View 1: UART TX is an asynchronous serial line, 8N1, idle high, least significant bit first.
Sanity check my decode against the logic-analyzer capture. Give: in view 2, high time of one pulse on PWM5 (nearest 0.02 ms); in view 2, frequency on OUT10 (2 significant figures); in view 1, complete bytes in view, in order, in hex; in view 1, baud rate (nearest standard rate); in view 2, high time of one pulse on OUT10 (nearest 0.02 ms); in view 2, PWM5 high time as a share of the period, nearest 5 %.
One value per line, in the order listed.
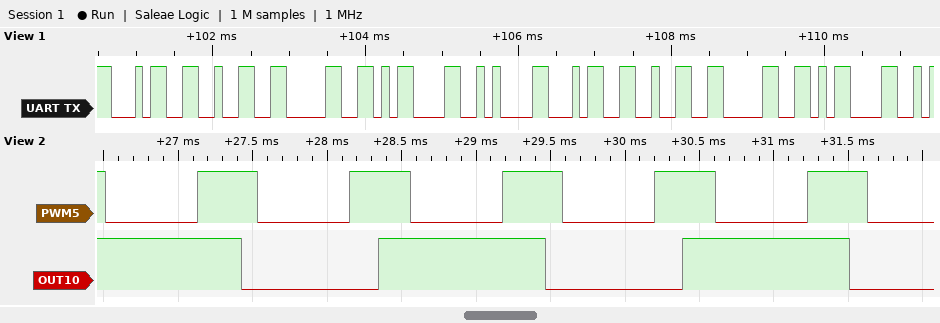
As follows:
0.40 ms
490 Hz
0x34 0x32 0x30 0x0D 0x0A 0x34 0x32 0x30 0x0D
9600 baud
1.12 ms
40 %
